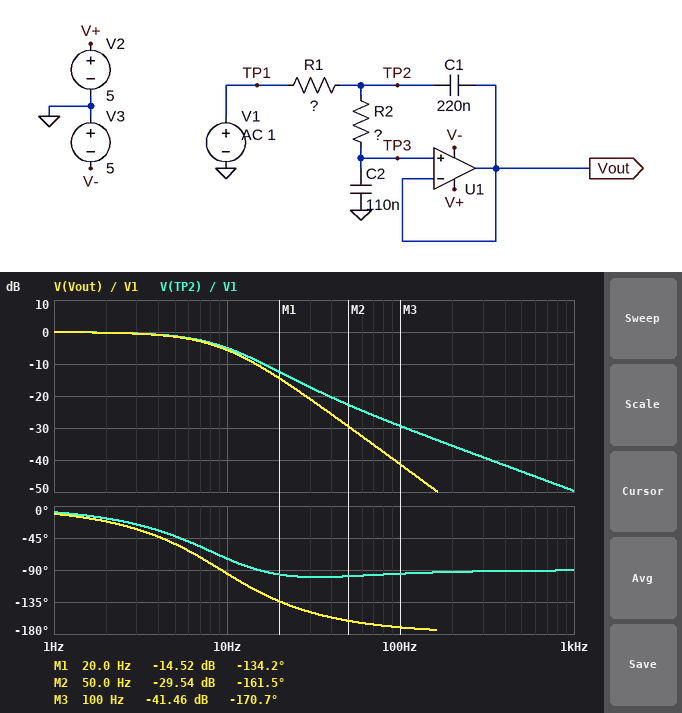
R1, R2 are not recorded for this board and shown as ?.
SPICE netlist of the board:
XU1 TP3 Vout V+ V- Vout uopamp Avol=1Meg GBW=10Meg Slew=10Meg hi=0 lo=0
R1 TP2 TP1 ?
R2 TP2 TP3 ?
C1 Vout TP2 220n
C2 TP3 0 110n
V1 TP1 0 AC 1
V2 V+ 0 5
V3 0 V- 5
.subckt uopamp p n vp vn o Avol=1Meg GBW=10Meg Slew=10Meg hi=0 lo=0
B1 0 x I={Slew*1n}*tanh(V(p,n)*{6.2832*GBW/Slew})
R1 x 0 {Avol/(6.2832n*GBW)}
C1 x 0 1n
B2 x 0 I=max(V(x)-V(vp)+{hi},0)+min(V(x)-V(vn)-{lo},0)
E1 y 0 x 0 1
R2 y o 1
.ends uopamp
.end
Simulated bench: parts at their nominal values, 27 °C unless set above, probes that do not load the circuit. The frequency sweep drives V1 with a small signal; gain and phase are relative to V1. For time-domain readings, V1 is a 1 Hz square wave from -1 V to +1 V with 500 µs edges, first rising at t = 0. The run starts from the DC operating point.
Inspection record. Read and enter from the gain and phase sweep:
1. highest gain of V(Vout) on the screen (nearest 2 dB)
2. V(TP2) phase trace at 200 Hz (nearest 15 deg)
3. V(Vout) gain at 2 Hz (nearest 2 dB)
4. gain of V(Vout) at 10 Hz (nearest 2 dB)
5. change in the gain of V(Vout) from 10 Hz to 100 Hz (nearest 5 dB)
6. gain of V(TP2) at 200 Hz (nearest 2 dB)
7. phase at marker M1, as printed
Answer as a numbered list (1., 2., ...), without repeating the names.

1. 0 dB
2. -90 deg
3. 0 dB
4. -6 dB
5. -35 dB
6. -36 dB
7. -134.2 deg
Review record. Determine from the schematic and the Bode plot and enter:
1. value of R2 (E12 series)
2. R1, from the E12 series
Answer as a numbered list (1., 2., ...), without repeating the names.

1. 56 kΩ
2. 220 kΩ
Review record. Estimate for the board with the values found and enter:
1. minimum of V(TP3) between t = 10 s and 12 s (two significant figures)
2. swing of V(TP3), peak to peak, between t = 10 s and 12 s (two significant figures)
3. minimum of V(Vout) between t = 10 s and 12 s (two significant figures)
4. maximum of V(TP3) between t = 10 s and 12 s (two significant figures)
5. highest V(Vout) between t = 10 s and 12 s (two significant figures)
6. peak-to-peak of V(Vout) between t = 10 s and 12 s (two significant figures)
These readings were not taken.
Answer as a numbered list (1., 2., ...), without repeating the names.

1. -1.0 V
2. 2.0 V
3. -1.0 V
4. 1.0 V
5. 1.0 V
6. 2.0 V
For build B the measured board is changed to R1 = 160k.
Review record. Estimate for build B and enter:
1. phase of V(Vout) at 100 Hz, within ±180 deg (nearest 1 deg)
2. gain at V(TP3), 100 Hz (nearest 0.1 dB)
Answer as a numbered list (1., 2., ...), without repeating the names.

1. -170 deg
2. -38.7 dB
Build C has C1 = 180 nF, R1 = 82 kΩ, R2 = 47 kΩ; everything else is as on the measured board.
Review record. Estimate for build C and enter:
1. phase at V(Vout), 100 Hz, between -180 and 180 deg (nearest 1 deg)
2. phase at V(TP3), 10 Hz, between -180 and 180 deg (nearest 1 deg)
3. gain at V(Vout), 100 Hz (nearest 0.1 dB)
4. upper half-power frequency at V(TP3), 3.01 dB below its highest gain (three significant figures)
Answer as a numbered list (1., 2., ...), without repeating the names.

1. -163 deg
2. -52 deg
3. -29.7 dB
4. 15.6 Hz
